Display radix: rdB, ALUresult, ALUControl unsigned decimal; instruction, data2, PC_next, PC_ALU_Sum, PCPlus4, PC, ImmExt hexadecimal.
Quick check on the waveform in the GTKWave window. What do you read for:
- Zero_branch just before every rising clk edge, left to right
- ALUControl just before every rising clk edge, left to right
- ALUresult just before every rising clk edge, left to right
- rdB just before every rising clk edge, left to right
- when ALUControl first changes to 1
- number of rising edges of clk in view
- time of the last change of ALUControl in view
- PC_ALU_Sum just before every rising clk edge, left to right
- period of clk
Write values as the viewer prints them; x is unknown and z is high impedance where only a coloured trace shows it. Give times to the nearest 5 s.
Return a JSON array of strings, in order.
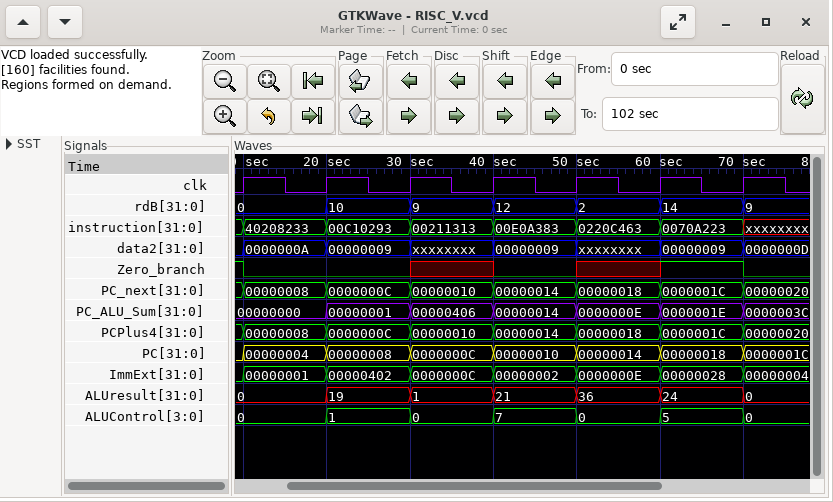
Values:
["1 0 0 x 0 x 1", "0, 0, 1, 0, 7, 0, 5", "0, 0, 19, 1, 21, 36, 24", "0, 0, 10, 9, 12, 2, 14", "20 s", "7", "70 s", "00000000, 00000000, 00000001, 00000406, 00000014, 0000000E, 0000001E", "10 s"]
